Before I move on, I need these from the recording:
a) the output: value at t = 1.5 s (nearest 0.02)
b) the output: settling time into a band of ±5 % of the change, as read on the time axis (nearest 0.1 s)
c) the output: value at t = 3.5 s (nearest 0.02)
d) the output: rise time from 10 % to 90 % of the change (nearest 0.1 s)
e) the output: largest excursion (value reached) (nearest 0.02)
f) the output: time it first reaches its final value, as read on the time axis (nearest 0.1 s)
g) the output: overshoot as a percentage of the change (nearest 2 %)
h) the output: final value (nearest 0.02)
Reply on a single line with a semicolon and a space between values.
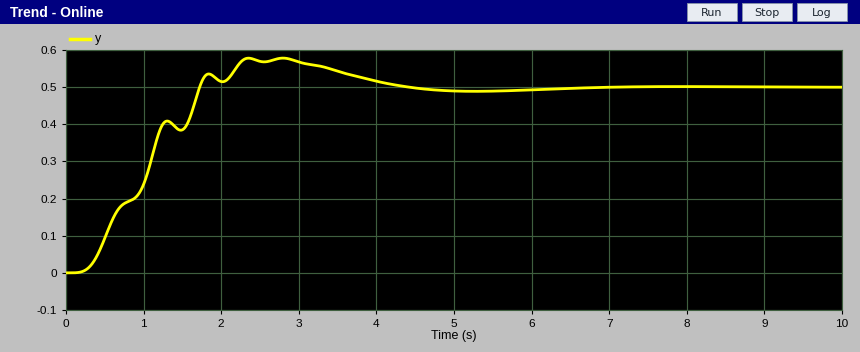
0.38; 3.8 s; 0.54; 1.2 s; 0.58; 1.7 s; 16 %; 0.50
